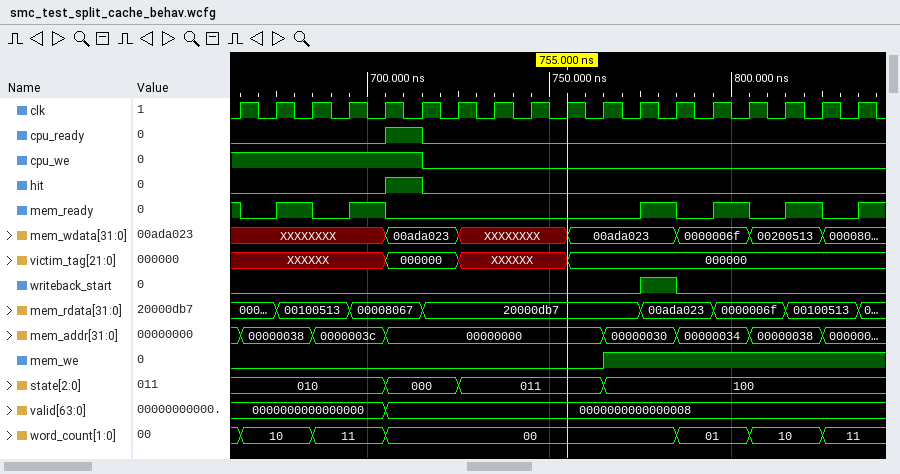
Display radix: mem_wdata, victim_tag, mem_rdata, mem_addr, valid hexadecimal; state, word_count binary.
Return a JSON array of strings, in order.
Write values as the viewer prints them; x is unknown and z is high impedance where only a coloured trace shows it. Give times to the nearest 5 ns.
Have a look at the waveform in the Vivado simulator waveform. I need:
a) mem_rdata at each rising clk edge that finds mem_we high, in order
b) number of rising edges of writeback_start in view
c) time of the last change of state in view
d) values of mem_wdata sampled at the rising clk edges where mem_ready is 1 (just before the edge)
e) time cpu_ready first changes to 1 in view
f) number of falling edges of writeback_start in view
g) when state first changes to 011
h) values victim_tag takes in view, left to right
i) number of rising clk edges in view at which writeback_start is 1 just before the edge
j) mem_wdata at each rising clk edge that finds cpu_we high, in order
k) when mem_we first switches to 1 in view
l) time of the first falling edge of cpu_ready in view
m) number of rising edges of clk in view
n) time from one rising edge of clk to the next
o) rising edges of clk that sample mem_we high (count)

["20000db7, 00ada023, 00ada023, 0000006f, 0000006f, 00100513, 00100513", "1", "765 ns", "XXXXXXXX, XXXXXXXX, XXXXXXXX, 00ada023, 0000006f, 00200513", "705 ns", "1", "725 ns", "XXXXXX, 000000, XXXXXX, 000000", "1", "XXXXXXXX, XXXXXXXX, XXXXXXXX, XXXXXXXX, XXXXXXXX, 00ada023", "765 ns", "715 ns", "18", "10 ns", "7"]
